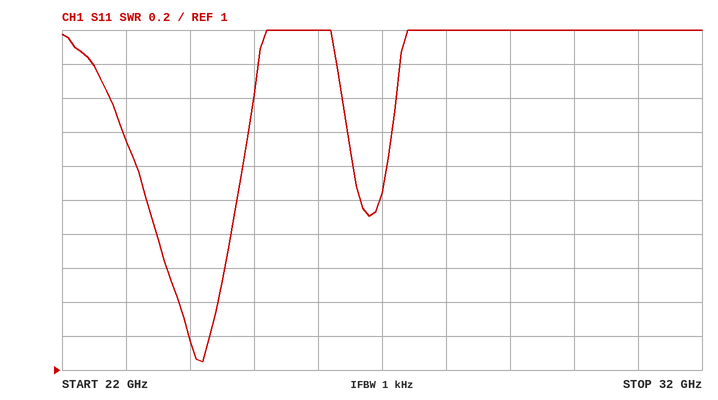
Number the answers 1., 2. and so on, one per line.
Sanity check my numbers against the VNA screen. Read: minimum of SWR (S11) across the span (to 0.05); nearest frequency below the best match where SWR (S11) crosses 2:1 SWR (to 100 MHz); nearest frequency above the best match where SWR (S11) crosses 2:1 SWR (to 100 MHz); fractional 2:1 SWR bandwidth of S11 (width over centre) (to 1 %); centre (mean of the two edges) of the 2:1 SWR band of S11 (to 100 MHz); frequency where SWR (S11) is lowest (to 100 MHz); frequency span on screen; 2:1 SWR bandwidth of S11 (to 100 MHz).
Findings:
1. 1.05
2. 23.3 GHz
3. 24.7 GHz
4. 6 %
5. 24.0 GHz
6. 24.2 GHz
7. 10 GHz
8. 1.4 GHz
